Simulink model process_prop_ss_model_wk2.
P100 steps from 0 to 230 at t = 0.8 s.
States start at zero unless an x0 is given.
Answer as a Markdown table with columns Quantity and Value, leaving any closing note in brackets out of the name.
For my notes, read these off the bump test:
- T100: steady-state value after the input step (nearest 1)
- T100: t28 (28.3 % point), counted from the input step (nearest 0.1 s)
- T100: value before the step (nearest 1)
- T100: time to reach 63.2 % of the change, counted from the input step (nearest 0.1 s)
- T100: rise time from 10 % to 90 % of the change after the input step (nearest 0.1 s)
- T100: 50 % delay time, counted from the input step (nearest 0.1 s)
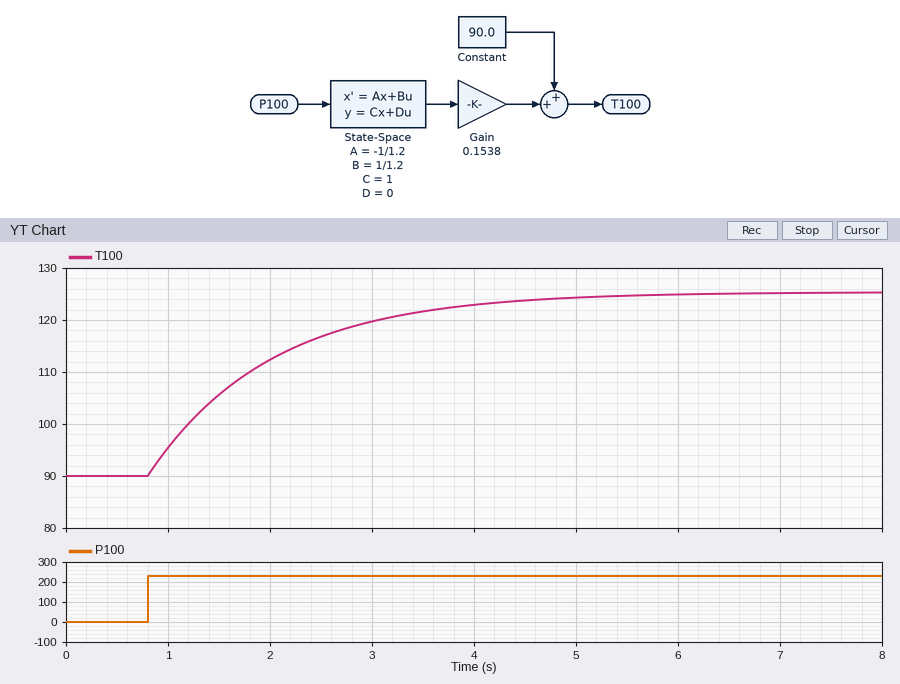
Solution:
| Quantity | Value |
|---|---|
| T100: steady-state value after the input step | 125 |
| T100: t28 (28.3 % point), counted from the input step | 0.4 s |
| T100: value before the step | 90 |
| T100: time to reach 63.2 % of the change, counted from the input step | 1.2 s |
| T100: rise time from 10 % to 90 % of the change after the input step | 2.6 s |
| T100: 50 % delay time, counted from the input step | 0.8 s |
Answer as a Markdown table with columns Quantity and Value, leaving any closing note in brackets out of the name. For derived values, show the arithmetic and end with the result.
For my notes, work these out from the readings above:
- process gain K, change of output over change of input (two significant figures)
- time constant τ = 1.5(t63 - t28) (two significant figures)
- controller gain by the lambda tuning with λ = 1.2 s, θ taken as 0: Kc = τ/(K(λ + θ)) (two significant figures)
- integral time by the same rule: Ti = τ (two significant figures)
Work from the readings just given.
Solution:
| Quantity | Value |
|---|---|
| process gain K, change of output over change of input | (125 - 90) / 230 = 0.15 |
| time constant τ = 1.5(t63 - t28) | 1.5 × (1.2 - 0.4) = 1.2 s |
| controller gain by the lambda tuning with λ = 1.2 s, θ taken as 0: Kc = τ/(K(λ + θ)) | 1.2 / (0.15 × (1.2 + 0)) = 6.7 |
| integral time by the same rule: Ti = τ | 1.2 s |
